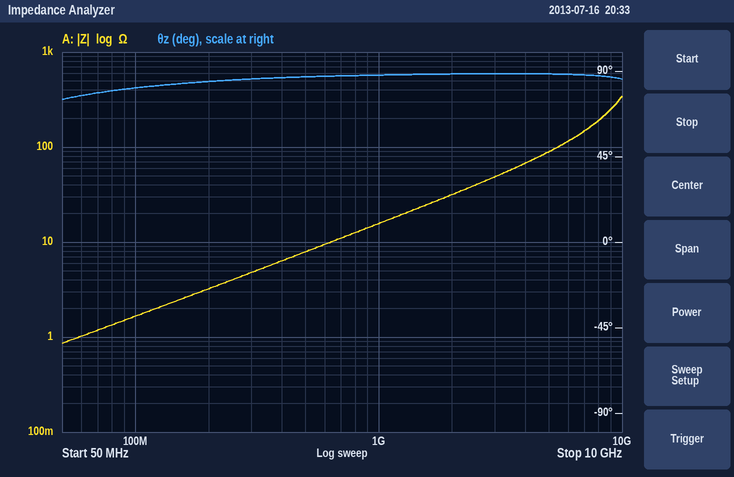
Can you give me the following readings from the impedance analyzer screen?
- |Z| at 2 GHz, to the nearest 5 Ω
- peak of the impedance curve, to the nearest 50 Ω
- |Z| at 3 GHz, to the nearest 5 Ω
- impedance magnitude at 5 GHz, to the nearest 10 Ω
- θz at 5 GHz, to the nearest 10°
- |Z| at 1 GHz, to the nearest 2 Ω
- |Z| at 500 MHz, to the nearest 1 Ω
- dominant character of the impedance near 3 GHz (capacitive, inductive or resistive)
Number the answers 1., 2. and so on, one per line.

1. 30 Ω
2. 350 Ω
3. 50 Ω
4. 90 Ω
5. 90°
6. 16 Ω
7. 8 Ω
8. inductive
